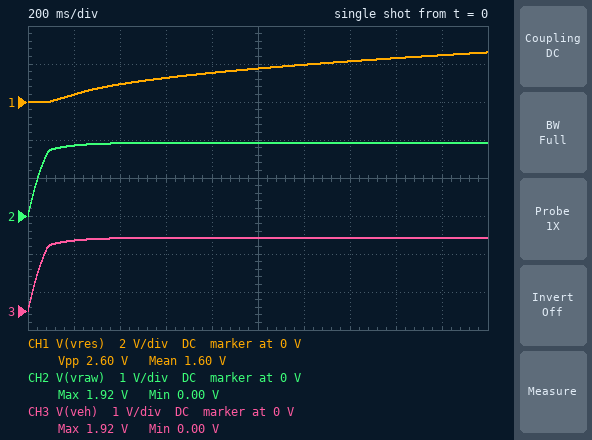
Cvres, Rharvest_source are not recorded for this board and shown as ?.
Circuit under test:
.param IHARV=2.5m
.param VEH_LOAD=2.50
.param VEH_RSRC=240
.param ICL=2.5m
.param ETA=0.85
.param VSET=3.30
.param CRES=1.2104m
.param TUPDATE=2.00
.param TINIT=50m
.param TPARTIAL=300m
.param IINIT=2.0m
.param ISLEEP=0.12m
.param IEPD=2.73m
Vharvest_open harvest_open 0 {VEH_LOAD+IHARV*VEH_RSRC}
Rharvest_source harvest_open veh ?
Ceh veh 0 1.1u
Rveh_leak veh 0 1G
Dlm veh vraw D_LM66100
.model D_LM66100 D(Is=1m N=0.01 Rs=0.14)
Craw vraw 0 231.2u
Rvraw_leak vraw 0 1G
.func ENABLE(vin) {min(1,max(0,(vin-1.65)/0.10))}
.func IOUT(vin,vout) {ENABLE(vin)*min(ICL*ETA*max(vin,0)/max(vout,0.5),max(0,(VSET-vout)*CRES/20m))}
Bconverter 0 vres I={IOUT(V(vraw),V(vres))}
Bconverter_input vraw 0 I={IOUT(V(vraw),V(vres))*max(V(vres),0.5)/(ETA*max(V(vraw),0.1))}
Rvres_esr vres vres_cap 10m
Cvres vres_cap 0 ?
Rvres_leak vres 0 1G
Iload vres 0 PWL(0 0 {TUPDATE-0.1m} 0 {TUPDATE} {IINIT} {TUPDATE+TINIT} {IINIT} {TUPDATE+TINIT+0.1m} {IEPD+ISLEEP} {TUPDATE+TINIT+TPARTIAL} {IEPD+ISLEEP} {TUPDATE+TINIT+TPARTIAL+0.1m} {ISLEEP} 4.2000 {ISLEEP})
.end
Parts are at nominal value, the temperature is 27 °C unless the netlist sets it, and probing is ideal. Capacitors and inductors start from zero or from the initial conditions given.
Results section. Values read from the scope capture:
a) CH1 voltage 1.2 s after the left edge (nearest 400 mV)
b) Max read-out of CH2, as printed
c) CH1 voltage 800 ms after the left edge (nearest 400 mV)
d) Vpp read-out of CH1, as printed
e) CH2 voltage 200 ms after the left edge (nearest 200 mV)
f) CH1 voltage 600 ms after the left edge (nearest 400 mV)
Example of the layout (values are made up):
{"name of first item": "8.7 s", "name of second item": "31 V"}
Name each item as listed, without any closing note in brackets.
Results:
{"CH1 voltage 1.2 s after the left edge": "2.0 V", "Max read-out of CH2, as printed": "1.92 V", "CH1 voltage 800 ms after the left edge": "1.6 V", "Vpp read-out of CH1, as printed": "2.60 V", "CH2 voltage 200 ms after the left edge": "1.8 V", "CH1 voltage 600 ms after the left edge": "1.2 V"}
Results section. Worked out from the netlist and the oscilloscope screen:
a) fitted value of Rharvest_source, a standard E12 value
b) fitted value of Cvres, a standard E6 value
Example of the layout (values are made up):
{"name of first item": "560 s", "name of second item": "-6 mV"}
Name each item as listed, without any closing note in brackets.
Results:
{"fitted value of Rharvest_source, a standard E12 value": "470 Ω", "fitted value of Cvres, a standard E6 value": "2.2 mF"}
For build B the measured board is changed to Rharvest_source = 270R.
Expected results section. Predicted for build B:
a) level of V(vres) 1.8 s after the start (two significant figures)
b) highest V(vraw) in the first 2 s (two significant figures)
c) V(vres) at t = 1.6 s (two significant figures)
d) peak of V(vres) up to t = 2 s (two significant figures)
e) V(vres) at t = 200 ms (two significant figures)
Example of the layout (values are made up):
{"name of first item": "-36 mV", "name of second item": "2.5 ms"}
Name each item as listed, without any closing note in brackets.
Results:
{"level of V(vres) 1.8 s after the start": "2.8 V", "highest V(vraw) in the first 2 s": "2.4 V", "V(vres) at t = 1.6 s": "2.6 V", "peak of V(vres) up to t = 2 s": "3.0 V", "V(vres) at t = 200 ms": "610 mV"}
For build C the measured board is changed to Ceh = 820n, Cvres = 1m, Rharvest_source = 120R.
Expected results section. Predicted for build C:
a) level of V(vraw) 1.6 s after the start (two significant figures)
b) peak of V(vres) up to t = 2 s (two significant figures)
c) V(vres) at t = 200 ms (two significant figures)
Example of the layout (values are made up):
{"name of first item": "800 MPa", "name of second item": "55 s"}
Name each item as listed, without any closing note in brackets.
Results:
{"level of V(vraw) 1.6 s after the start": "3.1 V", "peak of V(vres) up to t = 2 s": "3.3 V", "V(vres) at t = 200 ms": "1.3 V"}
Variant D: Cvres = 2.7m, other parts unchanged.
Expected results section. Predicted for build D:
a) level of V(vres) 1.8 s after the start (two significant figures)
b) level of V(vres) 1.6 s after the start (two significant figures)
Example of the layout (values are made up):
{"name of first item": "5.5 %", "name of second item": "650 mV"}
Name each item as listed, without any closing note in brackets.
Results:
{"level of V(vres) 1.8 s after the start": "2.2 V", "level of V(vres) 1.6 s after the start": "2.1 V"}
